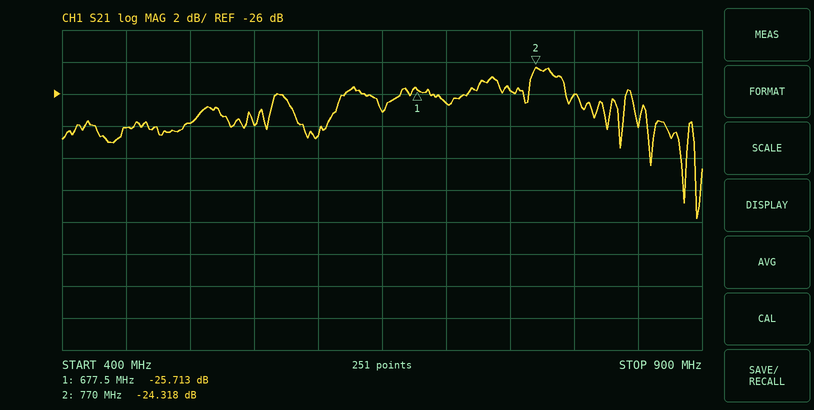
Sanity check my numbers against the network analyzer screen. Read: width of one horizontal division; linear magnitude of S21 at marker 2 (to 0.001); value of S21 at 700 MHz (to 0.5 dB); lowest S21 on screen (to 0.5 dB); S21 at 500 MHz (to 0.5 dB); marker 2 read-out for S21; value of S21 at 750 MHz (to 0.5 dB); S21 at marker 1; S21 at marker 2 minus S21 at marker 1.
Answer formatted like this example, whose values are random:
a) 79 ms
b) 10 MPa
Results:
a) 50 MHz
b) 0.061
c) -26.5 dB
d) -34.0 dB
e) -28.0 dB
f) -24.318 dB
g) -26.0 dB
h) -25.713 dB
i) 1.395 dB
